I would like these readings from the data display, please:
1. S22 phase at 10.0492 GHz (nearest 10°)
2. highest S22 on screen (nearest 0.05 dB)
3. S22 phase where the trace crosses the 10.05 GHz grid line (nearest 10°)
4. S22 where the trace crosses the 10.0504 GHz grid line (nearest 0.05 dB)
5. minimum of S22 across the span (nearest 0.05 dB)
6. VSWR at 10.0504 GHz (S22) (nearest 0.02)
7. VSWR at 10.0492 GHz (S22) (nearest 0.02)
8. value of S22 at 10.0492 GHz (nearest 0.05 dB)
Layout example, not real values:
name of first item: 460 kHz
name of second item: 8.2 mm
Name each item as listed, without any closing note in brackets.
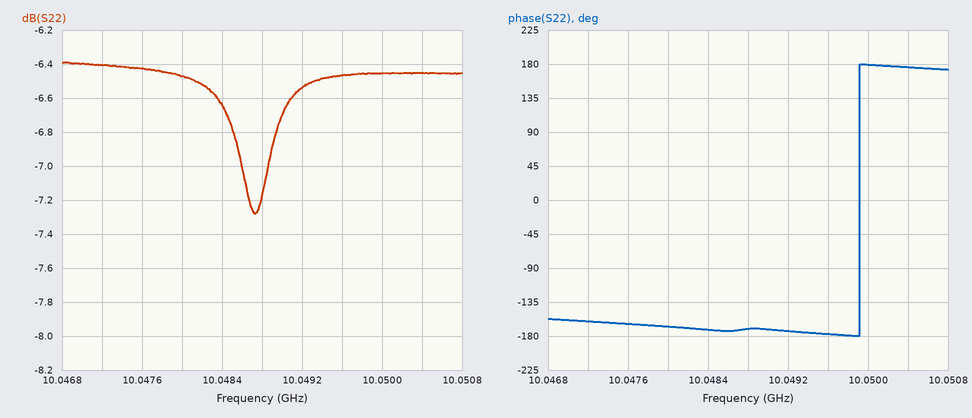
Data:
S22 phase at 10.0492 GHz: -170°
highest S22 on screen: -6.40 dB
S22 phase where the trace crosses the 10.05 GHz grid line: 180°
S22 where the trace crosses the 10.0504 GHz grid line: -6.45 dB
minimum of S22 across the span: -7.30 dB
VSWR at 10.0504 GHz (S22): 2.82
VSWR at 10.0492 GHz (S22): 2.78
value of S22 at 10.0492 GHz: -6.55 dB
